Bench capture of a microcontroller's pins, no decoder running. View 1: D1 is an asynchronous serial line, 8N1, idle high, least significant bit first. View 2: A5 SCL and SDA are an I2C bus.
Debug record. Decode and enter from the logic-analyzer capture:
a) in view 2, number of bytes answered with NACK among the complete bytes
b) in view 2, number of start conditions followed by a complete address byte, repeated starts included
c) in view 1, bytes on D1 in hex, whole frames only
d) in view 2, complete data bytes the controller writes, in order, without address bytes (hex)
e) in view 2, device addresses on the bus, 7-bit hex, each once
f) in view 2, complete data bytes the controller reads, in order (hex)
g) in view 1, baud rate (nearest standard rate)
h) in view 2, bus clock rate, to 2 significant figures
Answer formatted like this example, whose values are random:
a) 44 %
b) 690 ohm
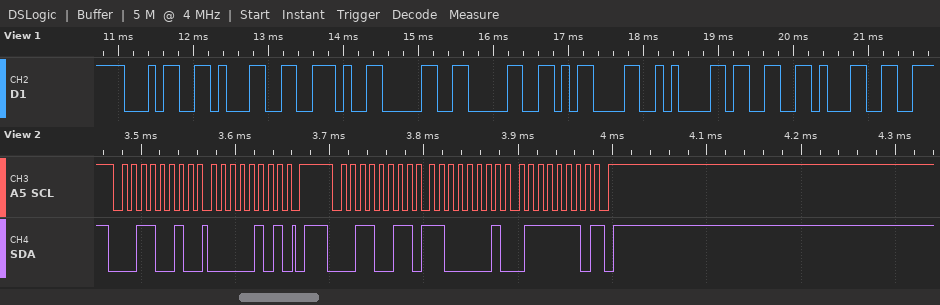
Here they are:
a) 1
b) 2
c) 34 31 2E 30 30 0D 0A 33 31
d) 05
e) 0x19
f) C1 7E
g) 9600 baud
h) 100 kHz
